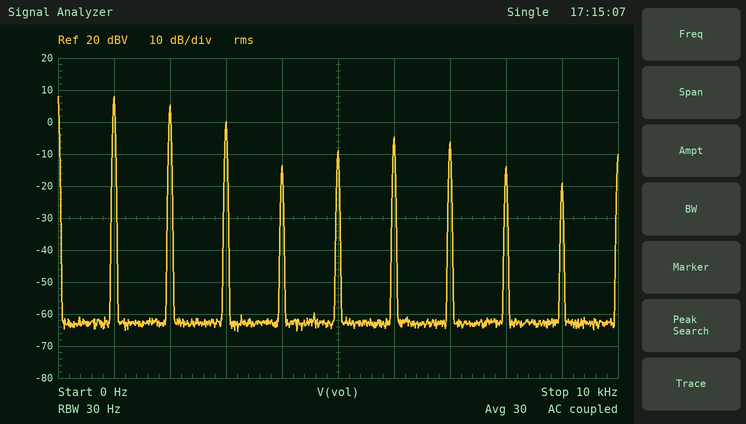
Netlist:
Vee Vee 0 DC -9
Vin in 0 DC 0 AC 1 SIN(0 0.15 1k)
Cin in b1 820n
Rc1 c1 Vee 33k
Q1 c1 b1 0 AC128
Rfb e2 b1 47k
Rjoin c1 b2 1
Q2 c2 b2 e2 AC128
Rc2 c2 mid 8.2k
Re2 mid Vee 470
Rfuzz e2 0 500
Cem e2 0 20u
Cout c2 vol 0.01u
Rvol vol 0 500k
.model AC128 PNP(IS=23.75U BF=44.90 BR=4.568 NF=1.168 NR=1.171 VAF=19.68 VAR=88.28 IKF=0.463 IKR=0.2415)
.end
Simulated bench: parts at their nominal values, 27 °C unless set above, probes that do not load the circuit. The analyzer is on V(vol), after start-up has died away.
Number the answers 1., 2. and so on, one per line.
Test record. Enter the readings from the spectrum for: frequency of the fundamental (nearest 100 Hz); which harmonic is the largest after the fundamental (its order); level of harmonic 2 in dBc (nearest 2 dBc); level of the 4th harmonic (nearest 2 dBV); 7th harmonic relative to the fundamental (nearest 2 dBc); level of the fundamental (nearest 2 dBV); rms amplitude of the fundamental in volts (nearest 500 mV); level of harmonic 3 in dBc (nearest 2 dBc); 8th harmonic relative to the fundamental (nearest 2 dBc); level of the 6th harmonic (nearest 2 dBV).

1. 1.0 kHz
2. 2
3. -2 dBc
4. -14 dBV
5. -14 dBc
6. 8 dBV
7. 2.5 V
8. -8 dBc
9. -22 dBc
10. -4 dBV
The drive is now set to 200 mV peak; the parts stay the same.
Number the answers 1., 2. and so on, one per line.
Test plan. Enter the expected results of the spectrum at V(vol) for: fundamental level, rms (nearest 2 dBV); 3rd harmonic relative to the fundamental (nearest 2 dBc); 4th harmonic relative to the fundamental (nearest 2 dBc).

1. 8 dBV
2. -6 dBc
3. -14 dBc
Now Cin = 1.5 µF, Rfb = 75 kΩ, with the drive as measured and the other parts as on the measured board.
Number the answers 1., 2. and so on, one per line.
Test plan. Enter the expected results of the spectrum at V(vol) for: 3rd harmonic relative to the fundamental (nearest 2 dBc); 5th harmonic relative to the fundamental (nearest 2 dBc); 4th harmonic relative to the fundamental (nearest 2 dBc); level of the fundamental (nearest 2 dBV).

1. -6 dBc
2. -22 dBc
3. -16 dBc
4. 8 dBV
